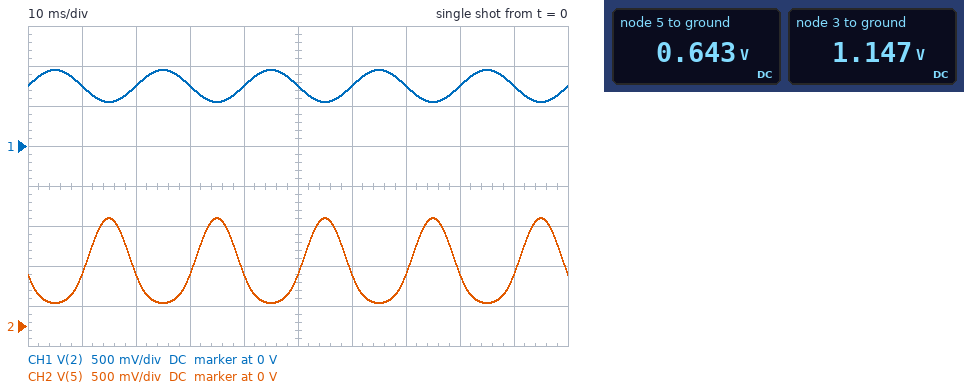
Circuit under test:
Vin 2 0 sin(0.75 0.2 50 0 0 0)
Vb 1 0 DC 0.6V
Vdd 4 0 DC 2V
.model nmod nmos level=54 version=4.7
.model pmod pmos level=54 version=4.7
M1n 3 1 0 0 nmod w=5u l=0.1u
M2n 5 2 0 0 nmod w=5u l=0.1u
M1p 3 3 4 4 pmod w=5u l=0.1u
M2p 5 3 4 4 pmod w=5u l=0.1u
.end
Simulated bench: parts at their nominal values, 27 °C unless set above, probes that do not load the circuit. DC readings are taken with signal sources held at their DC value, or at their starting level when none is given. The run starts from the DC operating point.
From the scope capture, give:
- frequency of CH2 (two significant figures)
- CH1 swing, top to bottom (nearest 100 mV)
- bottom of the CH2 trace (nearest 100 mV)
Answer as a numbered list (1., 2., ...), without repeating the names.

1. 50 Hz
2. 400 mV
3. 300 mV
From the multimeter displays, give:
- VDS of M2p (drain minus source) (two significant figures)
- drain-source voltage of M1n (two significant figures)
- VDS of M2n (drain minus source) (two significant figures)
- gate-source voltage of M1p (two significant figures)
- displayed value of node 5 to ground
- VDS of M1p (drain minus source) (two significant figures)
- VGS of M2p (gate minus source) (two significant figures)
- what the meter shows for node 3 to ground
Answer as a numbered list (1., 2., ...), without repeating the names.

1. -1.4 V
2. 1.1 V
3. 640 mV
4. -850 mV
5. 0.643 V
6. -850 mV
7. -850 mV
8. 1.147 V
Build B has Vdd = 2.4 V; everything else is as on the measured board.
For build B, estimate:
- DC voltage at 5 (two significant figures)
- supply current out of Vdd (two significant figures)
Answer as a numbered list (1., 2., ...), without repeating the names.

1. 940 mV
2. 2.9 mA
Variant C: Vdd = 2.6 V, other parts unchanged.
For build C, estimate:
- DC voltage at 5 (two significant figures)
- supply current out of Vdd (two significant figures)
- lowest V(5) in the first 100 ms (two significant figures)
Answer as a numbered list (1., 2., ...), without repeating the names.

1. 1.1 V
2. 3.1 mA
3. 570 mV
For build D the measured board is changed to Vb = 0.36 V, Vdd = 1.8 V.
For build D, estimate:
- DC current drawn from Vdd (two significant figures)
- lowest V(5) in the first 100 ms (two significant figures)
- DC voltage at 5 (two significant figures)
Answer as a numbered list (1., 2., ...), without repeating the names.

1. 610 µA
2. 47 mV
3. 69 mV
